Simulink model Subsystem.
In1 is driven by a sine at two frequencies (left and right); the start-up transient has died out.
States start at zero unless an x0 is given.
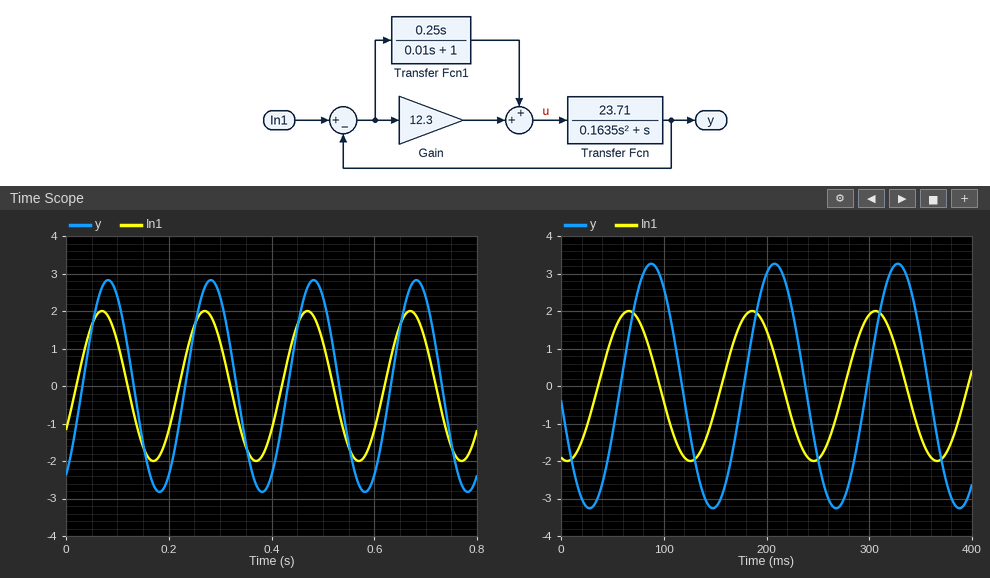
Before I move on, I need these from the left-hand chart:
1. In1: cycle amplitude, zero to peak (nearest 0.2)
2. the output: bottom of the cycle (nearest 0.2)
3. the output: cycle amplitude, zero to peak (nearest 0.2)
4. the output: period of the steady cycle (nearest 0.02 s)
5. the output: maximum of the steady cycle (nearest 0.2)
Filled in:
2.0
-2.8
2.8
0.20 s
2.8
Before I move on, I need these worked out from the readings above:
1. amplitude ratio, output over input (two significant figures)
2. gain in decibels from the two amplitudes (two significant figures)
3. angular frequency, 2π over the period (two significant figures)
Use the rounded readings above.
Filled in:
1.4
2.9 dB
31 rad/s
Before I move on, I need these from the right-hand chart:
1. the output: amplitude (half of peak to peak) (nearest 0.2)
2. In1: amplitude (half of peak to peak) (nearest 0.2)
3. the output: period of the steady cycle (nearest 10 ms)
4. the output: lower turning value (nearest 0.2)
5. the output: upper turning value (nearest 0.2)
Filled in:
3.2
2.0
120 ms
-3.2
3.2
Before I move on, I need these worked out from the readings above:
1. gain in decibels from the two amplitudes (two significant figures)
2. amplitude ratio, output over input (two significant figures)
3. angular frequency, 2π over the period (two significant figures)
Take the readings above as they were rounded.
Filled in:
4.1 dB
1.6
0.052 rad/ms
